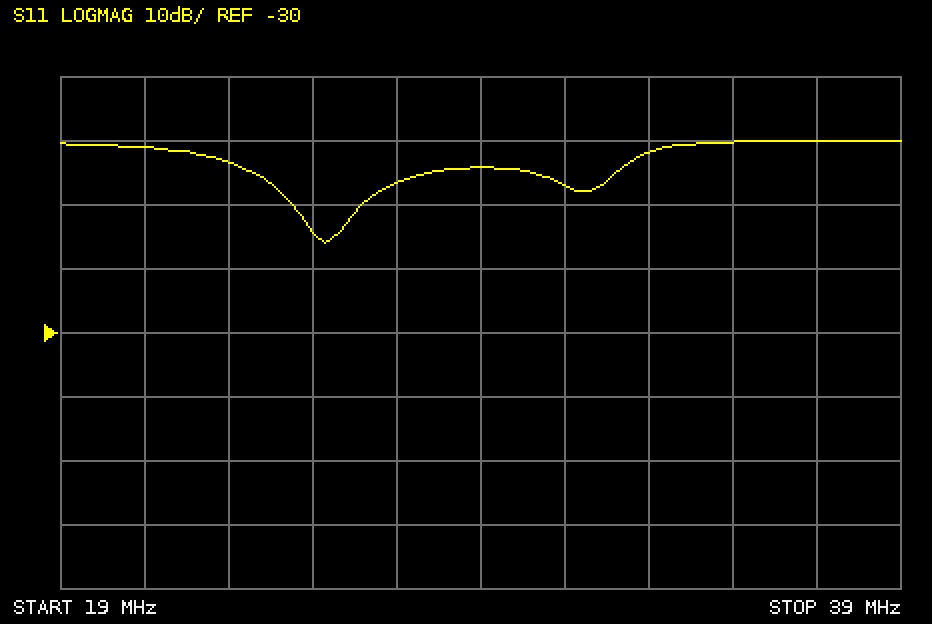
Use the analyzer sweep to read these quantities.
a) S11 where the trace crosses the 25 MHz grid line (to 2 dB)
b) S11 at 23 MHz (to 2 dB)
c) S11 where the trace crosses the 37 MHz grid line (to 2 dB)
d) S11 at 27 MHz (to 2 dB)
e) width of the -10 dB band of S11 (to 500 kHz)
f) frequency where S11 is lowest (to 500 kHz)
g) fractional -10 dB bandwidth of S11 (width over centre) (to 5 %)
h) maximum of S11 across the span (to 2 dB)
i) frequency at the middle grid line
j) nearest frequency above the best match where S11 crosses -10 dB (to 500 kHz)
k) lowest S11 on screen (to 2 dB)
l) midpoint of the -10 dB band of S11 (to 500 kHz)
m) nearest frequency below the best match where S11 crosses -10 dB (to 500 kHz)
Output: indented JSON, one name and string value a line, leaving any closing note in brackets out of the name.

{
  "S11 where the trace crosses the 25 MHz grid line": "-14 dB",
  "S11 at 23 MHz": "-4 dB",
  "S11 where the trace crosses the 37 MHz grid line": "0 dB",
  "S11 at 27 MHz": "-6 dB",
  "width of the -10 dB band of S11": "1.5 MHz",
  "frequency where S11 is lowest": "25.5 MHz",
  "fractional -10 dB bandwidth of S11 (width over centre)": "5 %",
  "maximum of S11 across the span": "0 dB",
  "frequency at the middle grid line": "29 MHz",
  "nearest frequency above the best match where S11 crosses -10 dB": "26.0 MHz",
  "lowest S11 on screen": "-16 dB",
  "midpoint of the -10 dB band of S11": "25.5 MHz",
  "nearest frequency below the best match where S11 crosses -10 dB": "24.5 MHz"
}
